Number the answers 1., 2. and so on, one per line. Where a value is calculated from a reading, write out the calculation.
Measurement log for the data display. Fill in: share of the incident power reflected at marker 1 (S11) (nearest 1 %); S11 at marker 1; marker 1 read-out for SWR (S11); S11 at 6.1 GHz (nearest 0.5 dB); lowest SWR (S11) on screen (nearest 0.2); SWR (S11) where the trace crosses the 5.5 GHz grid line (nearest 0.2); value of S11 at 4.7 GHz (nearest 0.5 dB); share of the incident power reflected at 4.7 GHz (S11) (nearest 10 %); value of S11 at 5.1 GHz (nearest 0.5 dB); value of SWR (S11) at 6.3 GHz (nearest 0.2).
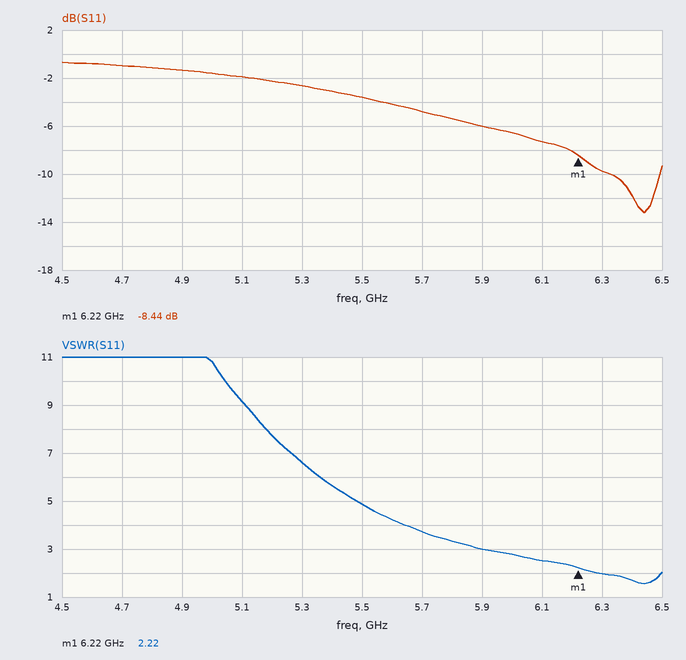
1. 10^(-8.44/10) ≈ 14 %
2. -8.44 dB
3. 2.22
4. -7.5 dB
5. 1.6
6. 4.8
7. -1.0 dB
8. 10^(-1/10) ≈ 79.4 %, so 80 % to the nearest 10 %
9. -2.0 dB
10. 2.0
